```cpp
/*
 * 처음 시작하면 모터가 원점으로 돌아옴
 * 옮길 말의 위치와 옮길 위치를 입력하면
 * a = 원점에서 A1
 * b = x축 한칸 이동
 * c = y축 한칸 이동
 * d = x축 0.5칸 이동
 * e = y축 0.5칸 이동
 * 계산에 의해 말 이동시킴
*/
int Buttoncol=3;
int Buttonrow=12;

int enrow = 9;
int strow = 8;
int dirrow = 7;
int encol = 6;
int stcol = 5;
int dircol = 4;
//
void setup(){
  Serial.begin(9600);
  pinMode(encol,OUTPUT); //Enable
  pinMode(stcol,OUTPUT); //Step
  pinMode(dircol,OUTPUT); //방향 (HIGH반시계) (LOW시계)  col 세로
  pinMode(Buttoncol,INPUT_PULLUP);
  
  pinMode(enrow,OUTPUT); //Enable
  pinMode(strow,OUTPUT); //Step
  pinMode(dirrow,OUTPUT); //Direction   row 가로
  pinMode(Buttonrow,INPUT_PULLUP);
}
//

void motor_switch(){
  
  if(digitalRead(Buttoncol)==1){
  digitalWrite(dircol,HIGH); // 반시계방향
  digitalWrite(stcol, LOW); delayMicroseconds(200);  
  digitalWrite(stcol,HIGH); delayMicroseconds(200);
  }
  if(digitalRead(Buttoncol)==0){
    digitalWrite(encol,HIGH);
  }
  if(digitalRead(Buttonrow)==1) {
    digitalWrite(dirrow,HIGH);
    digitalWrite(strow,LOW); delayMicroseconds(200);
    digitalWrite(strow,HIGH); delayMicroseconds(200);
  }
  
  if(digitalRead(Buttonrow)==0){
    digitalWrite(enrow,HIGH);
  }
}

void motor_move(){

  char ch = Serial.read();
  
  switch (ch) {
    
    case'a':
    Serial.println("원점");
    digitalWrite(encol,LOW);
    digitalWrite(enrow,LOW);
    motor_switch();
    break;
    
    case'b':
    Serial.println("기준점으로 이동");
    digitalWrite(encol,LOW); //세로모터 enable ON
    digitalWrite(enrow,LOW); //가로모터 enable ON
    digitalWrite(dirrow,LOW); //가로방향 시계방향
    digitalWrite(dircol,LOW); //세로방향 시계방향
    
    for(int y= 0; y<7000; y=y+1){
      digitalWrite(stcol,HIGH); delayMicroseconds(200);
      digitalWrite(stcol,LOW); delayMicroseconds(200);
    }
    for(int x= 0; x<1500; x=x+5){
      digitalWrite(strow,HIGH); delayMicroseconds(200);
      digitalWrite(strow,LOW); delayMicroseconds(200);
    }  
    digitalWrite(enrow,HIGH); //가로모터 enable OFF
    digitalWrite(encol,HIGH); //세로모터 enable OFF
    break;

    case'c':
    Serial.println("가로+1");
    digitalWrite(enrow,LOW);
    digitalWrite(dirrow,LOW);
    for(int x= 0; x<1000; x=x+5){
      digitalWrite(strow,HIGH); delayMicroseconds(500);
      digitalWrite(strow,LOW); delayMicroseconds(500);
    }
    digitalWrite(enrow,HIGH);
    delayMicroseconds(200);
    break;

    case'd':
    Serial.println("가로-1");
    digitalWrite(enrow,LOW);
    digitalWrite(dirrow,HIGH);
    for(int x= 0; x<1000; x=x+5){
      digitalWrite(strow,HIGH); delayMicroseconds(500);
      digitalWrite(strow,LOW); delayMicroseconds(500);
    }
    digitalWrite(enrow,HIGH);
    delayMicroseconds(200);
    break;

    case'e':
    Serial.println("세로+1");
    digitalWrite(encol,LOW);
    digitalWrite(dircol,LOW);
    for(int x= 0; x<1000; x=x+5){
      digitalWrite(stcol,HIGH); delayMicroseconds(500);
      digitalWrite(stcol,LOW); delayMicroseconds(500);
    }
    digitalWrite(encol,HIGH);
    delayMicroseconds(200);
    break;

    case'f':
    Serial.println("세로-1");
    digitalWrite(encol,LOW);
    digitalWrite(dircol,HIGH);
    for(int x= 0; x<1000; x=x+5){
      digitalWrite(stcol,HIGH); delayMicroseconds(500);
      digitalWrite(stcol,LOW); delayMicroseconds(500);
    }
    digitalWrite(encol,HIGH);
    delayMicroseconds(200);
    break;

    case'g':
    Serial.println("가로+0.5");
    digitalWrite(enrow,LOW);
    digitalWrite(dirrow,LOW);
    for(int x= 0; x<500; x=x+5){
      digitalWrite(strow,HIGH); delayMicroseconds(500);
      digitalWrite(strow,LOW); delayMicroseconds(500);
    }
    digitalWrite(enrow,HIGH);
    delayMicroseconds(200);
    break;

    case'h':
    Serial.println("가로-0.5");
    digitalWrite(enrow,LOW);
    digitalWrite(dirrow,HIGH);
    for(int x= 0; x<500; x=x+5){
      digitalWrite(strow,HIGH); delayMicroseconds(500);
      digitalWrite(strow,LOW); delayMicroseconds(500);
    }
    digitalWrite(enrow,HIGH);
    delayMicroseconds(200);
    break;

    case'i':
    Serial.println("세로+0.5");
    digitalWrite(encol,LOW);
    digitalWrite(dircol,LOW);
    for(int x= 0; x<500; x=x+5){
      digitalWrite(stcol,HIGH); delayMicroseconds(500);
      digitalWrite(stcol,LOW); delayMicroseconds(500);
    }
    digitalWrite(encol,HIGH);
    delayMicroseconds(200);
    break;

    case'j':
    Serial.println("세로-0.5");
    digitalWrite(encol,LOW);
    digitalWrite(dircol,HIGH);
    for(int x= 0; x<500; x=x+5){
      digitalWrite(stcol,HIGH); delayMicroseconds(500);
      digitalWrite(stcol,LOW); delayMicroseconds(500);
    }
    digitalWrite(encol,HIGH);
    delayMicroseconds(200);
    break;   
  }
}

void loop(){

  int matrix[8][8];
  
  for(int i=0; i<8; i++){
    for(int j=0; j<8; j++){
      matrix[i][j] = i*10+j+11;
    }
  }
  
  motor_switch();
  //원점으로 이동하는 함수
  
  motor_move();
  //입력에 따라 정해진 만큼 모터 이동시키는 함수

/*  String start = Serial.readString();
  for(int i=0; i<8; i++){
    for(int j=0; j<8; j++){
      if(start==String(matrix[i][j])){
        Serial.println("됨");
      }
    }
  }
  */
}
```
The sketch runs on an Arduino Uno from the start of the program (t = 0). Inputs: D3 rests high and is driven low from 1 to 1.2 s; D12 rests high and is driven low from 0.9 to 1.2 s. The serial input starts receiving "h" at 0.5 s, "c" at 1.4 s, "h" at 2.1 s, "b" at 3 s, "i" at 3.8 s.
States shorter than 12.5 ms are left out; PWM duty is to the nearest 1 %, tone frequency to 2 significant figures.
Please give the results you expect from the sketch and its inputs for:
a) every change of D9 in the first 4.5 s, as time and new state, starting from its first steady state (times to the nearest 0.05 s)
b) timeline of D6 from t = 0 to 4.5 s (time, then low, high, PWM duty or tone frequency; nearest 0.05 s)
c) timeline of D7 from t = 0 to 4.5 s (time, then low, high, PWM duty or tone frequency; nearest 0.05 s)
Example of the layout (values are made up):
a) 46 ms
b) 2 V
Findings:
a) 0 s low; 0.6 s high; 1.4 s low; 1.6 s high; 2.1 s low; 2.2 s high; 3 s low
b) 0 s low; 1 s high; 3 s low
c) 0 s high; 1.4 s low; 1.6 s high; 3 s low
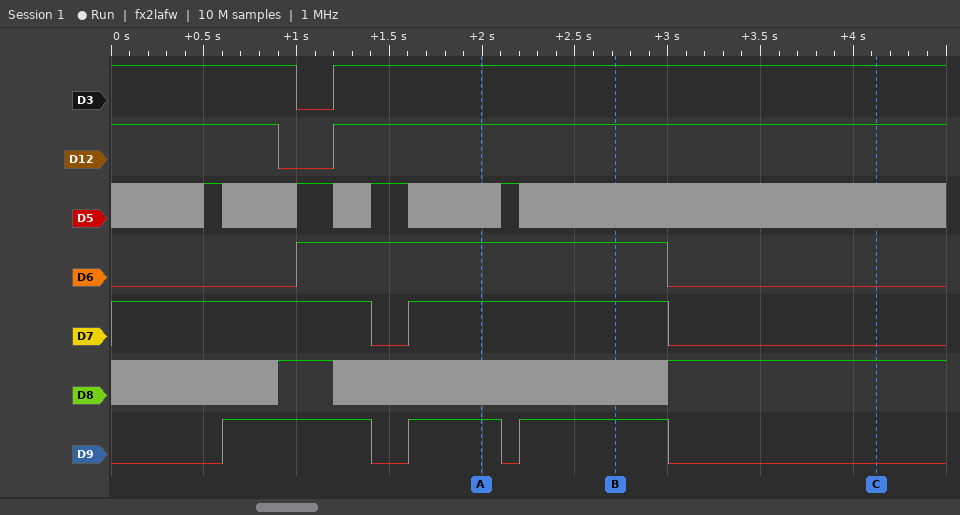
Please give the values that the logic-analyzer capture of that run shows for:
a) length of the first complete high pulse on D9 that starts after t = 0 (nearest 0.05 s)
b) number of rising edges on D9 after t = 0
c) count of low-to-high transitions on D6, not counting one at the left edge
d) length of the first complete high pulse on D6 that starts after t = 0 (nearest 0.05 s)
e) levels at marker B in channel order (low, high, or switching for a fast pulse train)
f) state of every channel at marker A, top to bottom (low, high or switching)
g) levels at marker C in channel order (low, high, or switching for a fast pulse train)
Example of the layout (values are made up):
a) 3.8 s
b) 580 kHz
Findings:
a) 0.80 s
b) 3
c) 1
d) 2.00 s
e) D3 high, D12 high, D5 switching, D6 high, D7 high, D8 switching, D9 high
f) D3 high, D12 high, D5 switching, D6 high, D7 high, D8 switching, D9 high
g) D3 high, D12 high, D5 switching, D6 low, D7 low, D8 high, D9 low
